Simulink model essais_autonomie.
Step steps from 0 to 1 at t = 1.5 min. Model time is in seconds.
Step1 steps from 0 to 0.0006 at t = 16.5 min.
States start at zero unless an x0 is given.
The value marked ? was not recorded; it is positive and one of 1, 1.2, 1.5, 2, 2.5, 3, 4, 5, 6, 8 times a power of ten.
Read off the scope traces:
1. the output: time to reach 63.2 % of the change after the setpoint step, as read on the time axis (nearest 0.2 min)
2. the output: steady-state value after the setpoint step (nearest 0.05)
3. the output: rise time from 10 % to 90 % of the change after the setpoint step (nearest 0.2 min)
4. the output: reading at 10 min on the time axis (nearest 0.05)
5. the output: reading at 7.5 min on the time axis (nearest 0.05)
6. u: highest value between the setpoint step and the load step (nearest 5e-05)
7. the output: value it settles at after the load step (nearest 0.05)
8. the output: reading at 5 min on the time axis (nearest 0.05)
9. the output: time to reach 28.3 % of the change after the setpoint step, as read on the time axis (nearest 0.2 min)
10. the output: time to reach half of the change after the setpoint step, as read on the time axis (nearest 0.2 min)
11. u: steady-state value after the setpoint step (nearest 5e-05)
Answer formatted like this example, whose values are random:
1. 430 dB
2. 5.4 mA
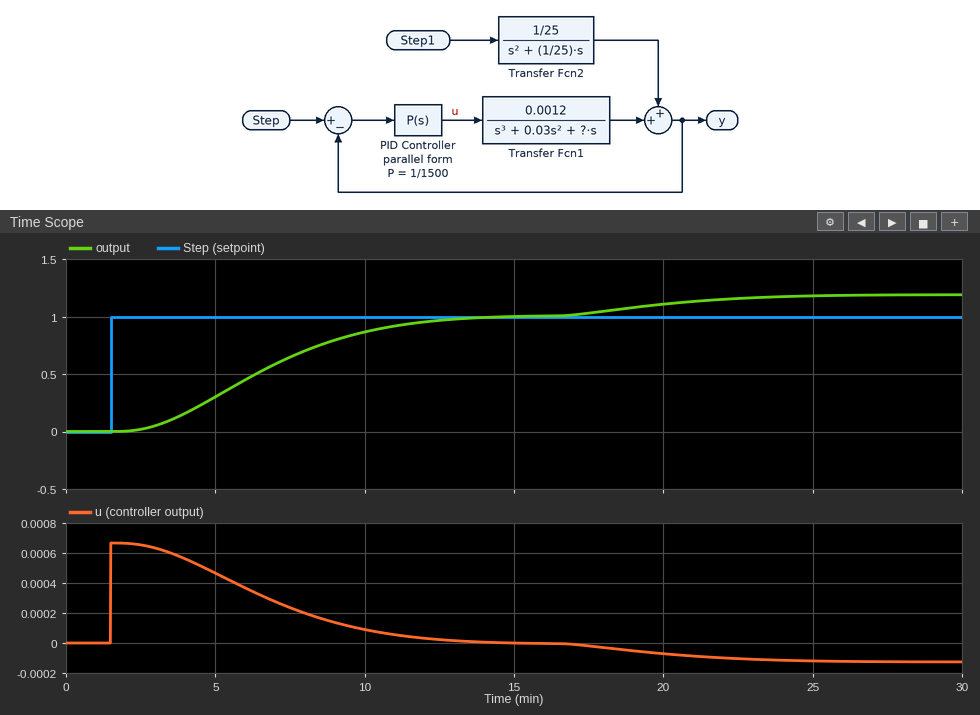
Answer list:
1. 7.4 min
2. 1.00
3. 7.2 min
4. 0.85
5. 0.65
6. 0.00065
7. 1.20
8. 0.30
9. 4.8 min
10. 6.4 min
11. 0.00000
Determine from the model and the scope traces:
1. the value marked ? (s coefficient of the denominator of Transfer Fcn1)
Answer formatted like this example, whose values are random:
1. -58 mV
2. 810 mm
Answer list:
1. 0.00025
